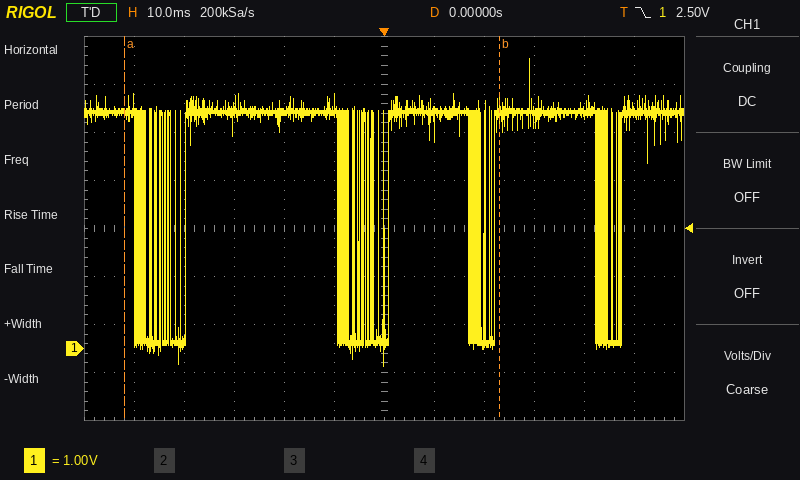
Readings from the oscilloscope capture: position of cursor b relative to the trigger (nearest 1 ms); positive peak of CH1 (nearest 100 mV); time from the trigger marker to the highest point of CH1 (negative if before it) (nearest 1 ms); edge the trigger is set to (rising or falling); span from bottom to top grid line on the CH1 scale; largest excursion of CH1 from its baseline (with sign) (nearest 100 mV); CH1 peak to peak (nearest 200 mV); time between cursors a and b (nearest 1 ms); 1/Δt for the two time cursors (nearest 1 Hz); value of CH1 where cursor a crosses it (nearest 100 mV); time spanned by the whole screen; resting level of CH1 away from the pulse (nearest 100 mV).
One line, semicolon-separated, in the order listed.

+23 ms; 6.0 V; +29 ms; falling; 8 V; -5.3 V; 6.4 V; 75 ms; 13 Hz; 4.9 V; 120 ms; 4.9 V
